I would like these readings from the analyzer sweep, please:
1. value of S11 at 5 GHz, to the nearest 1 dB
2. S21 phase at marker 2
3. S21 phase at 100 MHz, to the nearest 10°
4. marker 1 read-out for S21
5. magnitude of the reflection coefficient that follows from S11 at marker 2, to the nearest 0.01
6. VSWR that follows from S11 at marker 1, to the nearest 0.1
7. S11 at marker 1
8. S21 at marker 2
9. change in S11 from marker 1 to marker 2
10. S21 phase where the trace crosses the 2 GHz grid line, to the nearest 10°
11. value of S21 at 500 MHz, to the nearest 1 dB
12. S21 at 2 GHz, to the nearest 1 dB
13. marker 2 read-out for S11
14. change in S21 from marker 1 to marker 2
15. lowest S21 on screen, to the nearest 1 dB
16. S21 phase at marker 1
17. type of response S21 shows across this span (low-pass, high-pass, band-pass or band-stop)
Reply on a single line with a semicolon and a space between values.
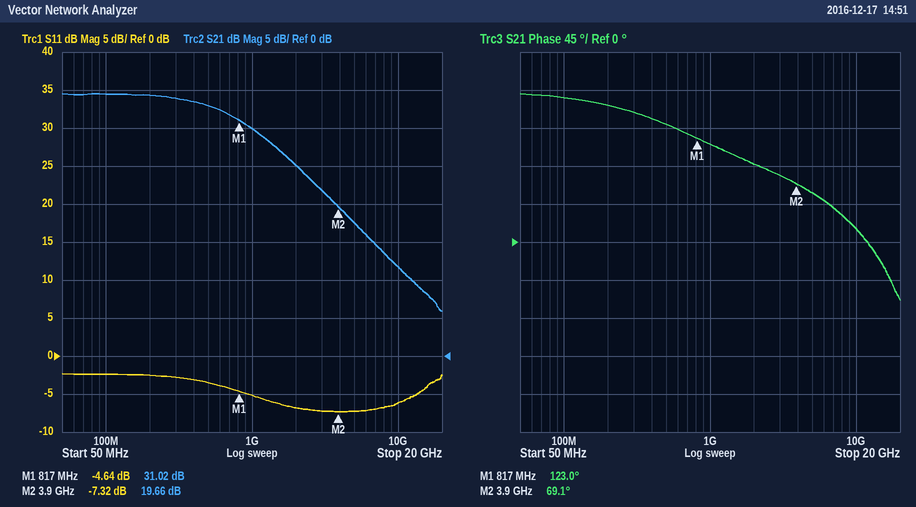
-7 dB; 69.1°; 170°; 31.02 dB; 0.43; 3.8; -4.64 dB; 19.66 dB; -2.68 dB; 90°; 33 dB; 25 dB; -7.32 dB; -11.36 dB; 6 dB; 123.0°; low-pass
